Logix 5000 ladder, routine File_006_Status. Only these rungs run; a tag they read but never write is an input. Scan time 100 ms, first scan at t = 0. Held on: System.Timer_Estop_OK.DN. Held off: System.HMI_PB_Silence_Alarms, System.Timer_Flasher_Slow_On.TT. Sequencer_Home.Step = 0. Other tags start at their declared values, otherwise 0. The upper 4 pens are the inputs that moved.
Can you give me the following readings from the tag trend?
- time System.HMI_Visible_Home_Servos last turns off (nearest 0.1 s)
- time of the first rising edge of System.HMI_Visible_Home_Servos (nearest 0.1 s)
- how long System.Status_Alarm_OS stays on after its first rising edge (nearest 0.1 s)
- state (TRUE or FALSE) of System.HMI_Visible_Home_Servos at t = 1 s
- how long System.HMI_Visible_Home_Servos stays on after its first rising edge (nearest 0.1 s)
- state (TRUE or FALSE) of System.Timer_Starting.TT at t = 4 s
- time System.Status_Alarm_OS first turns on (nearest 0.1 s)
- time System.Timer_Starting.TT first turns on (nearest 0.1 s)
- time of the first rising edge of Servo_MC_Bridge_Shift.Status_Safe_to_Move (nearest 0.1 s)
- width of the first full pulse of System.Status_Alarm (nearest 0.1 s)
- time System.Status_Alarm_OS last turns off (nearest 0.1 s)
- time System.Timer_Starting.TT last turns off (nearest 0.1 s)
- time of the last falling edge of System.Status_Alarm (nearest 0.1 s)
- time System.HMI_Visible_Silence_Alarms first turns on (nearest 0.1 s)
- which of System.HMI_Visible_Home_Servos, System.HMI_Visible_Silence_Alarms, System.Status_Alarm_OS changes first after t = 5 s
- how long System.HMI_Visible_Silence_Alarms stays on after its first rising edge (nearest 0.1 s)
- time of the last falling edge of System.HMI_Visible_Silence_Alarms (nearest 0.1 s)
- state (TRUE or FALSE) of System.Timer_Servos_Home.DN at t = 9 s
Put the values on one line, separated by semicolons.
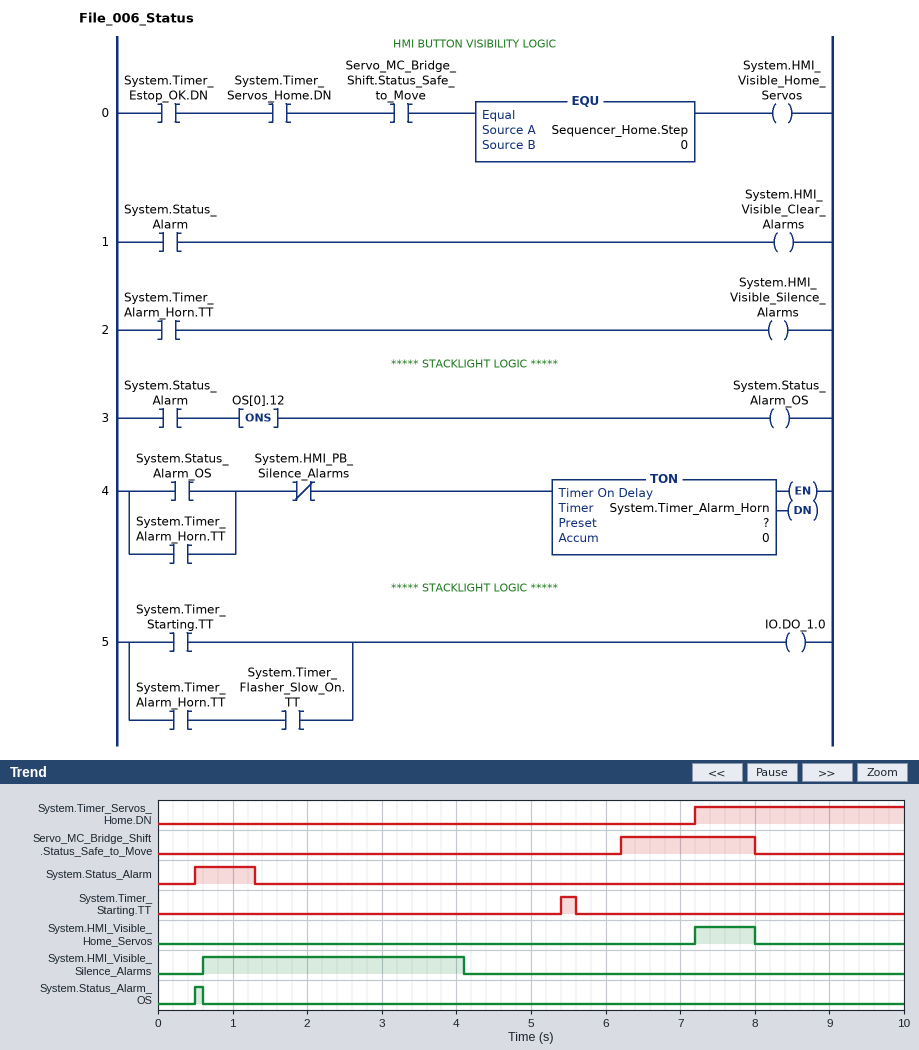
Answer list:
8.0 s; 7.2 s; 0.1 s; FALSE; 0.8 s; FALSE; 0.5 s; 5.4 s; 6.2 s; 0.8 s; 0.6 s; 5.6 s; 1.3 s; 0.6 s; System.HMI_Visible_Home_Servos; 3.5 s; 4.1 s; TRUE
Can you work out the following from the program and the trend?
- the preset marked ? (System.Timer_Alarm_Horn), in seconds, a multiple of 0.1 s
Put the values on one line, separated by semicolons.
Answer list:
3.5 s
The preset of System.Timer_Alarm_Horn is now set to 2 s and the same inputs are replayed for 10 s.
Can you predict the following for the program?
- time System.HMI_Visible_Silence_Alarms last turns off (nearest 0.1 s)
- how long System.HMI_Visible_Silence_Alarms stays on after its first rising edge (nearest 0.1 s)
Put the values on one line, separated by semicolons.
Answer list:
2.6 s; 2.0 s
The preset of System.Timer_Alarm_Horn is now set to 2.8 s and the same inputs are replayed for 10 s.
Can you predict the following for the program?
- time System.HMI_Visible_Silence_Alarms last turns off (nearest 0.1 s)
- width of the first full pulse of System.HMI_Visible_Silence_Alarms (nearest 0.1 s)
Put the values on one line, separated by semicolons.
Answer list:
3.4 s; 2.8 s
